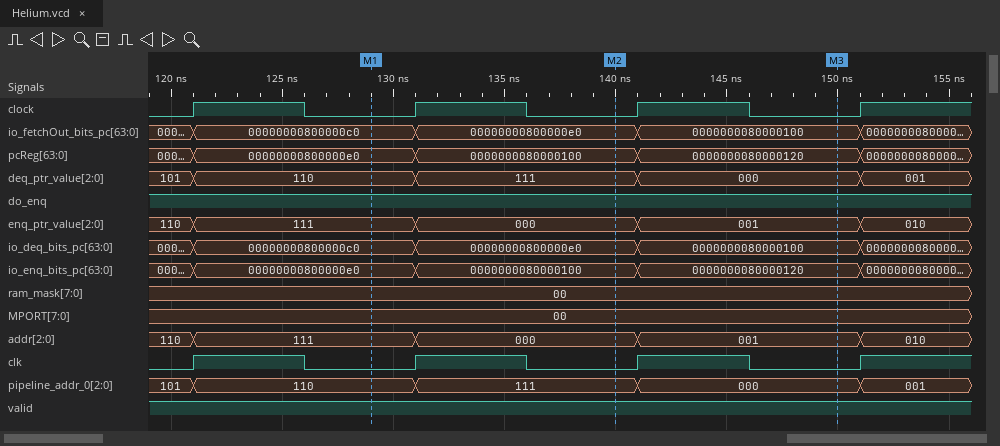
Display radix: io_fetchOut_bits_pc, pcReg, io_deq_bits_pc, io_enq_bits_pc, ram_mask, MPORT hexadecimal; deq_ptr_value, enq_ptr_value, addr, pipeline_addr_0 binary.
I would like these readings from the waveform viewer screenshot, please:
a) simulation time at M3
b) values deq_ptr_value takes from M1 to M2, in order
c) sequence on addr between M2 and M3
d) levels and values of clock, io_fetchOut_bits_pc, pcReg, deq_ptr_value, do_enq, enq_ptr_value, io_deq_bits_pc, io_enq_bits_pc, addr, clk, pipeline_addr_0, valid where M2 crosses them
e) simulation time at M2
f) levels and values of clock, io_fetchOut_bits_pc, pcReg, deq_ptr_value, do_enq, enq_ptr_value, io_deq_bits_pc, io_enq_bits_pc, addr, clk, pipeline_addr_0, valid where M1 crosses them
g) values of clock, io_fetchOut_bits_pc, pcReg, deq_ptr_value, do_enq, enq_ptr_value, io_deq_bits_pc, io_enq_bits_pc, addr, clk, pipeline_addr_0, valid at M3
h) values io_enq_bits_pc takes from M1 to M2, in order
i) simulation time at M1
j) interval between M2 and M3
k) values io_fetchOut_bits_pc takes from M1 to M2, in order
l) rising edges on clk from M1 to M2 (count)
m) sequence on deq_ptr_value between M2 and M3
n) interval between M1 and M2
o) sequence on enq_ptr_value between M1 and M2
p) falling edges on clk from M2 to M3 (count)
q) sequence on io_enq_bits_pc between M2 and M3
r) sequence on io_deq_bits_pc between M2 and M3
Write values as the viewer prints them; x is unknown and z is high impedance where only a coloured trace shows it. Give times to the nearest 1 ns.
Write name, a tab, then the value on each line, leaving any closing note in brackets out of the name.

simulation time at M3	150 ns
values deq_ptr_value takes from M1 to M2, in order	110, 111
sequence on addr between M2 and M3	000, 001
levels and values of clock, io_fetchOut_bits_pc, pcReg, deq_ptr_value, do_enq, enq_ptr_value, io_deq_bits_pc, io_enq_bits_pc, addr, clk, pipeline_addr_0, valid where M2 crosses them	clock=0, io_fetchOut_bits_pc=00000000800000e0, pcReg=0000000080000100, deq_ptr_value=111, do_enq=1, enq_ptr_value=000, io_deq_bits_pc=00000000800000e0, io_enq_bits_pc=0000000080000100, addr=000, clk=0, pipeline_addr_0=111, valid=1
simulation time at M2	140 ns
levels and values of clock, io_fetchOut_bits_pc, pcReg, deq_ptr_value, do_enq, enq_ptr_value, io_deq_bits_pc, io_enq_bits_pc, addr, clk, pipeline_addr_0, valid where M1 crosses them	clock=0, io_fetchOut_bits_pc=00000000800000c0, pcReg=00000000800000e0, deq_ptr_value=110, do_enq=1, enq_ptr_value=111, io_deq_bits_pc=00000000800000c0, io_enq_bits_pc=00000000800000e0, addr=111, clk=0, pipeline_addr_0=110, valid=1
values of clock, io_fetchOut_bits_pc, pcReg, deq_ptr_value, do_enq, enq_ptr_value, io_deq_bits_pc, io_enq_bits_pc, addr, clk, pipeline_addr_0, valid at M3	clock=0, io_fetchOut_bits_pc=0000000080000100, pcReg=0000000080000120, deq_ptr_value=000, do_enq=1, enq_ptr_value=001, io_deq_bits_pc=0000000080000100, io_enq_bits_pc=0000000080000120, addr=001, clk=0, pipeline_addr_0=000, valid=1
values io_enq_bits_pc takes from M1 to M2, in order	00000000800000e0, 0000000080000100
simulation time at M1	129 ns
interval between M2 and M3	10 ns
values io_fetchOut_bits_pc takes from M1 to M2, in order	00000000800000c0, 00000000800000e0
rising edges on clk from M1 to M2	1
sequence on deq_ptr_value between M2 and M3	111, 000
interval between M1 and M2	11 ns
sequence on enq_ptr_value between M1 and M2	111, 000
falling edges on clk from M2 to M3	1
sequence on io_enq_bits_pc between M2 and M3	0000000080000100, 0000000080000120
sequence on io_deq_bits_pc between M2 and M3	00000000800000e0, 0000000080000100
